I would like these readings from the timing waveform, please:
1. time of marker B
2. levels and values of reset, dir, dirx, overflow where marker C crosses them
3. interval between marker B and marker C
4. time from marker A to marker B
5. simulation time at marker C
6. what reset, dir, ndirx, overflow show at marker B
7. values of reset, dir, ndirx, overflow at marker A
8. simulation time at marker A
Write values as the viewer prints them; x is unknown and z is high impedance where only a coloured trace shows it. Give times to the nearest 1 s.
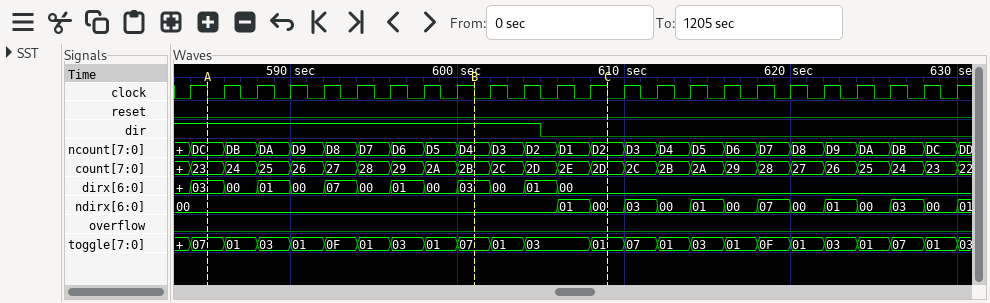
601 s
reset=0, dir=0, dirx=00, overflow=0
8 s
16 s
609 s
reset=0, dir=1, ndirx=00, overflow=0
reset=0, dir=1, ndirx=00, overflow=0
585 s
